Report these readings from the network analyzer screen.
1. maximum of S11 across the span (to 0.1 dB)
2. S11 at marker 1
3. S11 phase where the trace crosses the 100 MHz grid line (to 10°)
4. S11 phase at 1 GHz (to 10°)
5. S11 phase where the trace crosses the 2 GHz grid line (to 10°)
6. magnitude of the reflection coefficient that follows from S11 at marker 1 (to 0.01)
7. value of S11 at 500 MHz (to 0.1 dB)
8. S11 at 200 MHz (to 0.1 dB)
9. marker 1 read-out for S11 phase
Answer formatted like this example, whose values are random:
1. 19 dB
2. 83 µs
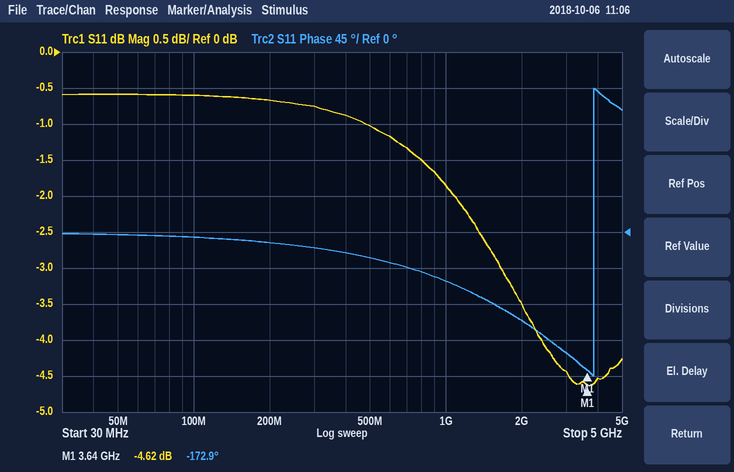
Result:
1. -0.6 dB
2. -4.62 dB
3. -10°
4. -60°
5. -110°
6. 0.59
7. -1.0 dB
8. -0.7 dB
9. -172.9°
